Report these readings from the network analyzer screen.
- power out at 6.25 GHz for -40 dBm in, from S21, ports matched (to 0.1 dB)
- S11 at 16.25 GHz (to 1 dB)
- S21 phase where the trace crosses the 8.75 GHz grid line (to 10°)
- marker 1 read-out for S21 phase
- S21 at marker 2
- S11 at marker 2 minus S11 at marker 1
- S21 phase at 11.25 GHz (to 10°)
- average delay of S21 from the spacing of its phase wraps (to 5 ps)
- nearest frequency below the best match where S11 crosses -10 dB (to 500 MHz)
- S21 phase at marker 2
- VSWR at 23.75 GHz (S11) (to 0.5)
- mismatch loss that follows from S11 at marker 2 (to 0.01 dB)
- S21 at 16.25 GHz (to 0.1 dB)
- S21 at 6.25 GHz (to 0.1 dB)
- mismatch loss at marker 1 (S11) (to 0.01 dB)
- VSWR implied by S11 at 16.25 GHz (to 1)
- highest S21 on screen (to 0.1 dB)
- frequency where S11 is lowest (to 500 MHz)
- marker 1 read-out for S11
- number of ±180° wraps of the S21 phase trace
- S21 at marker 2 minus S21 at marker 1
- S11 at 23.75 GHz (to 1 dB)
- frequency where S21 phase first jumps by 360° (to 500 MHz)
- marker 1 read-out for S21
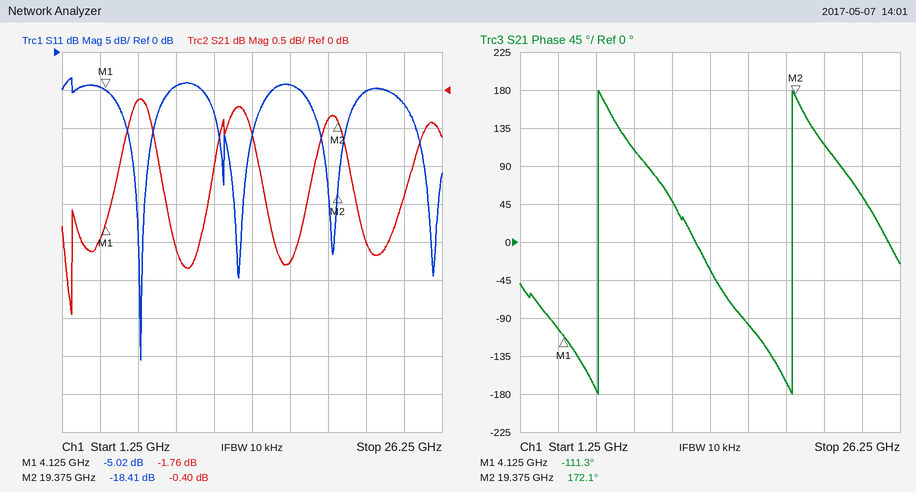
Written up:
-40.1 dBm
-4 dB
110°
-111.3°
-0.40 dB
-13.39 dB
50°
80 ps
5.5 GHz
172.1°
2.5
0.06 dB
-2.3 dB
-0.1 dB
1.64 dB
4
-0.1 dB
6.5 GHz
-5.02 dB
2
1.36 dB
-7 dB
6.5 GHz
-1.76 dB
